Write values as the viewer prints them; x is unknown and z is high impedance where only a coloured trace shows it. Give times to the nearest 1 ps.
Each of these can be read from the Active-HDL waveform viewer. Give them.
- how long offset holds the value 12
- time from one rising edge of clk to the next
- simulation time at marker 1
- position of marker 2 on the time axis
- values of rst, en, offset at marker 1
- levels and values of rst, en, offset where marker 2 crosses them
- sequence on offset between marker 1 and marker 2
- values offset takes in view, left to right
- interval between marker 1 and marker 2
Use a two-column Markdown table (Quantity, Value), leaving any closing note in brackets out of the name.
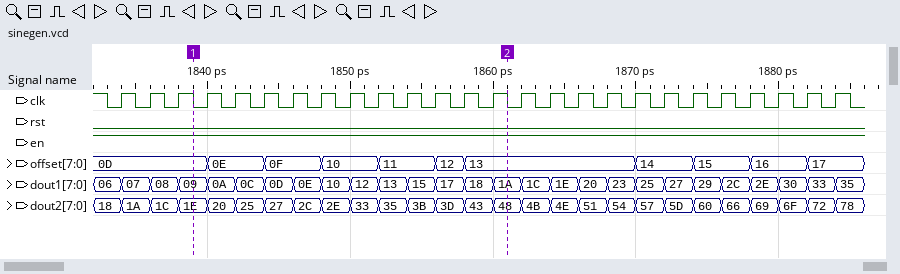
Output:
| Quantity | Value |
|---|---|
| how long offset holds the value 12 | 2 ps |
| time from one rising edge of clk to the next | 2 ps |
| simulation time at marker 1 | 1839 ps |
| position of marker 2 on the time axis | 1861 ps |
| values of rst, en, offset at marker 1 | rst=0, en=1, offset=0D |
| levels and values of rst, en, offset where marker 2 crosses them | rst=0, en=1, offset=13 |
| sequence on offset between marker 1 and marker 2 | 0D, 0E, 0F, 10, 11, 12, 13 |
| values offset takes in view, left to right | 0D, 0E, 0F, 10, 11, 12, 13, 14, 15, 16, 17 |
| interval between marker 1 and marker 2 | 22 ps |
